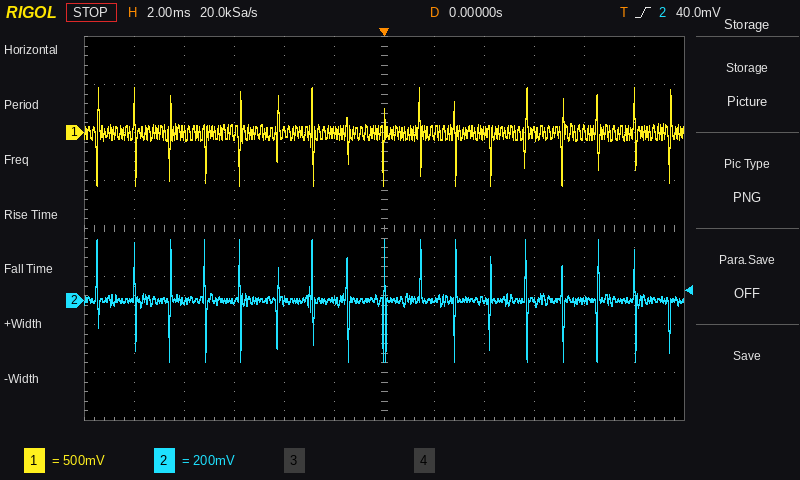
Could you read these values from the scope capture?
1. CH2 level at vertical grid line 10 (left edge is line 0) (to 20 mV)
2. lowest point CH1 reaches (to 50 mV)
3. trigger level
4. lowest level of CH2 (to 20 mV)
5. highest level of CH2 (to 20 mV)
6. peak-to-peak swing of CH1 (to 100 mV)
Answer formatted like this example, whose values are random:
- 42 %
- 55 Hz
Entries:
- 0 mV
- -550 mV
- 40.0 mV
- -260 mV
- 260 mV
- 1.00 V
